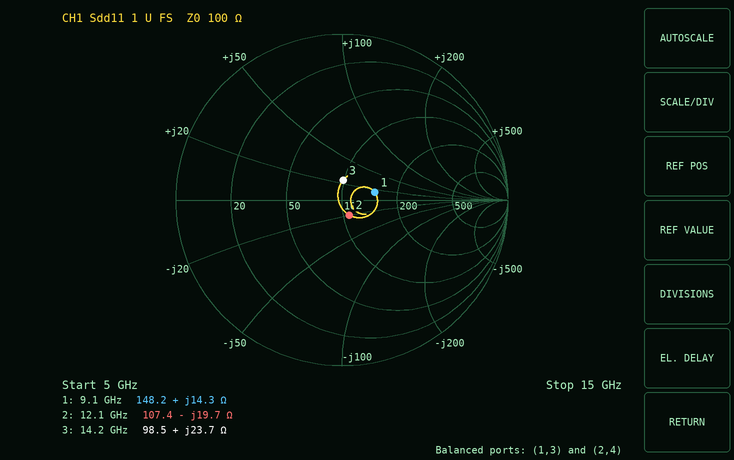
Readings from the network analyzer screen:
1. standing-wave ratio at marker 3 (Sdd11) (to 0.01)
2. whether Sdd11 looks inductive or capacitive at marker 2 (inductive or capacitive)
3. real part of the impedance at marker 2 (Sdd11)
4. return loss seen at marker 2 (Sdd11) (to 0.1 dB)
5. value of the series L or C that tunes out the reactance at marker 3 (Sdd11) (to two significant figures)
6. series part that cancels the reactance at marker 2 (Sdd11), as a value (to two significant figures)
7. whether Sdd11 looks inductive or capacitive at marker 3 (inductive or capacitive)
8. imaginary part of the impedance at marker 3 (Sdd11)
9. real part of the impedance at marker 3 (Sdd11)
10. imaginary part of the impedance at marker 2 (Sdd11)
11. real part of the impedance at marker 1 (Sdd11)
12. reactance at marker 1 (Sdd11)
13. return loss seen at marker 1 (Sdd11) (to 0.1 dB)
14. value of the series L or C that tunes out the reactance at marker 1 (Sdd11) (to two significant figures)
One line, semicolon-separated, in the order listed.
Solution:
1.27; capacitive; 107.4 Ω; 19.9 dB; 470 fF; 260 pH; inductive; +23.7 Ω; 98.5 Ω; -19.7 Ω; 148.2 Ω; +14.3 Ω; 13.9 dB; 1.2 pF
